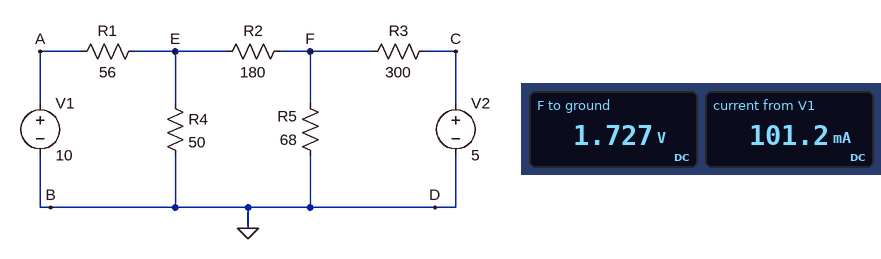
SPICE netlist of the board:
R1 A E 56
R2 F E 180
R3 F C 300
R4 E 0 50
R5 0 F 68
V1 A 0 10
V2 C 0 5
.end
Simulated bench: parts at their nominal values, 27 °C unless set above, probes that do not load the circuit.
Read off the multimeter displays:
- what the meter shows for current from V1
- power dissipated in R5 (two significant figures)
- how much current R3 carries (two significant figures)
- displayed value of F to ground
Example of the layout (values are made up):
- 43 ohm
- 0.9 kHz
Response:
- 101.2 mA
- 44 mW
- 11 mA
- 1.727 V
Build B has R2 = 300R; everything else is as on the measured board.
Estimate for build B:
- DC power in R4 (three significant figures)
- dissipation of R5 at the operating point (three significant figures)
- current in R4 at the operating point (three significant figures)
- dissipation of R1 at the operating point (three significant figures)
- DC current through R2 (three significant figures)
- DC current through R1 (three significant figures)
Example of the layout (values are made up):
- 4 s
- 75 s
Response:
- 397 mW
- 32.0 mW
- 89.1 mA
- 549 mW
- 9.93 mA
- 99.0 mA
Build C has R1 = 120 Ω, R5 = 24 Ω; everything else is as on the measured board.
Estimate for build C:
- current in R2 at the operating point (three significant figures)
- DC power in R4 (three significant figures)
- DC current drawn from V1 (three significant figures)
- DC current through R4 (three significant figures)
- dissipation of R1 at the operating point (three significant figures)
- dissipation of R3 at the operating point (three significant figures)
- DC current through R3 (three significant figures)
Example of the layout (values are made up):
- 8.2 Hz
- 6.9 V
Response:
- 10.8 mA
- 131 mW
- 62.0 mA
- 51.2 mA
- 461 mW
- 64.2 mW
- 14.6 mA
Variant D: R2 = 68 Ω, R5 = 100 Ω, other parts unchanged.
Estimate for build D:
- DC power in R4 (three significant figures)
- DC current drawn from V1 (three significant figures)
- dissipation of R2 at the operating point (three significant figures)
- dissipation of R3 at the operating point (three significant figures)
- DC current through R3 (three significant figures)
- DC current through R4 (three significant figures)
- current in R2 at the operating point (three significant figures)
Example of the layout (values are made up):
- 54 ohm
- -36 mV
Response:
- 349 mW
- 104 mA
- 28.5 mW
- 16.4 mW
- 7.38 mA
- 83.5 mA
- 20.5 mA
